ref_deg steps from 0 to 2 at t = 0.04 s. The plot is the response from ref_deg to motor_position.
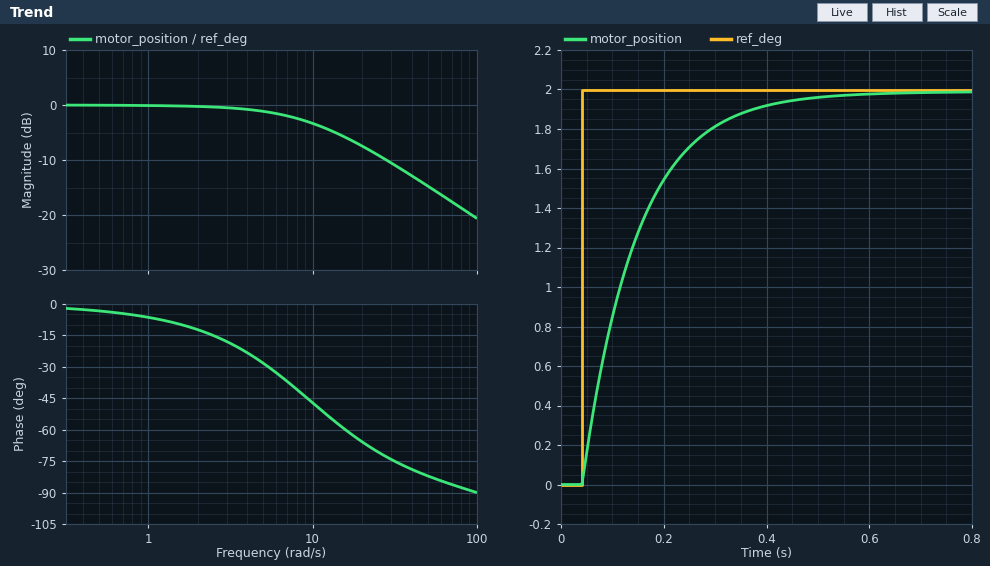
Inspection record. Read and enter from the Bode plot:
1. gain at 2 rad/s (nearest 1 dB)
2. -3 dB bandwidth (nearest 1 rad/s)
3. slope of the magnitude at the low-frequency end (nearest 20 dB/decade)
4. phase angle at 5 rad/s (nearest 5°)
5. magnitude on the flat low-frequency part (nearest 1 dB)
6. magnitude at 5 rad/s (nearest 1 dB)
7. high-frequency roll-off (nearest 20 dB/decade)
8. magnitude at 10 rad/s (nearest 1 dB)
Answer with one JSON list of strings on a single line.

["0 dB", "9 rad/s", "0 dB/decade", "-30°", "0 dB", "-1 dB", "-20 dB/decade", "-3 dB"]
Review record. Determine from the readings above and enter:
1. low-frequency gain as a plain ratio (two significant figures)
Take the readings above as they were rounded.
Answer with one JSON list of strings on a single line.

["1.0"]
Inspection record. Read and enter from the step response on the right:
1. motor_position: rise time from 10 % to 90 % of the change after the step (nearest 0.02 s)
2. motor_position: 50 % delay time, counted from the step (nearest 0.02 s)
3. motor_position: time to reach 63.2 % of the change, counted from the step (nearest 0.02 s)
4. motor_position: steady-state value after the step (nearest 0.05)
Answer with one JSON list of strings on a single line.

["0.24 s", "0.08 s", "0.10 s", "2.00"]
